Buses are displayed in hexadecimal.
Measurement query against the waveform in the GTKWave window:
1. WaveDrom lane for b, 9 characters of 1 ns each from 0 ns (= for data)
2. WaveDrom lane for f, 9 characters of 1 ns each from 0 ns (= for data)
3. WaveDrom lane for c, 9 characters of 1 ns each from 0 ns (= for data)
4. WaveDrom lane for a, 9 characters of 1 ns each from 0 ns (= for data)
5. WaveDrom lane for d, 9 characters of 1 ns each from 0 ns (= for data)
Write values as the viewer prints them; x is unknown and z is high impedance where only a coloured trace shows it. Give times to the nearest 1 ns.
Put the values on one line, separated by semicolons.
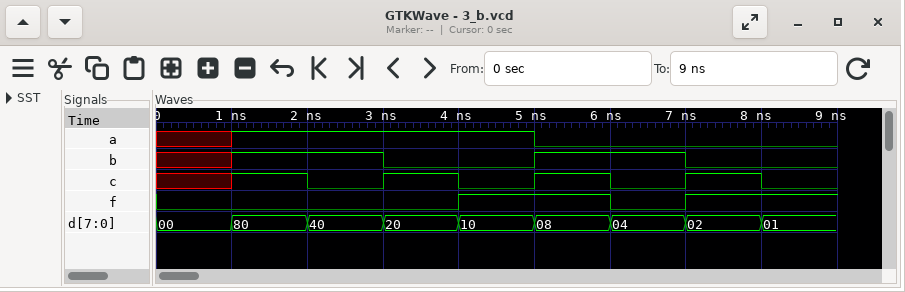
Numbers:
{name: 'b', wave: 'x1.0.1.0.'}; {name: 'f', wave: '0...1.01.'}; {name: 'c', wave: 'x10101010'}; {name: 'a', wave: 'x1...0...'}; {name: 'd', wave: '=========', data: '00 80 40 20 10 08 04 02 01'}
